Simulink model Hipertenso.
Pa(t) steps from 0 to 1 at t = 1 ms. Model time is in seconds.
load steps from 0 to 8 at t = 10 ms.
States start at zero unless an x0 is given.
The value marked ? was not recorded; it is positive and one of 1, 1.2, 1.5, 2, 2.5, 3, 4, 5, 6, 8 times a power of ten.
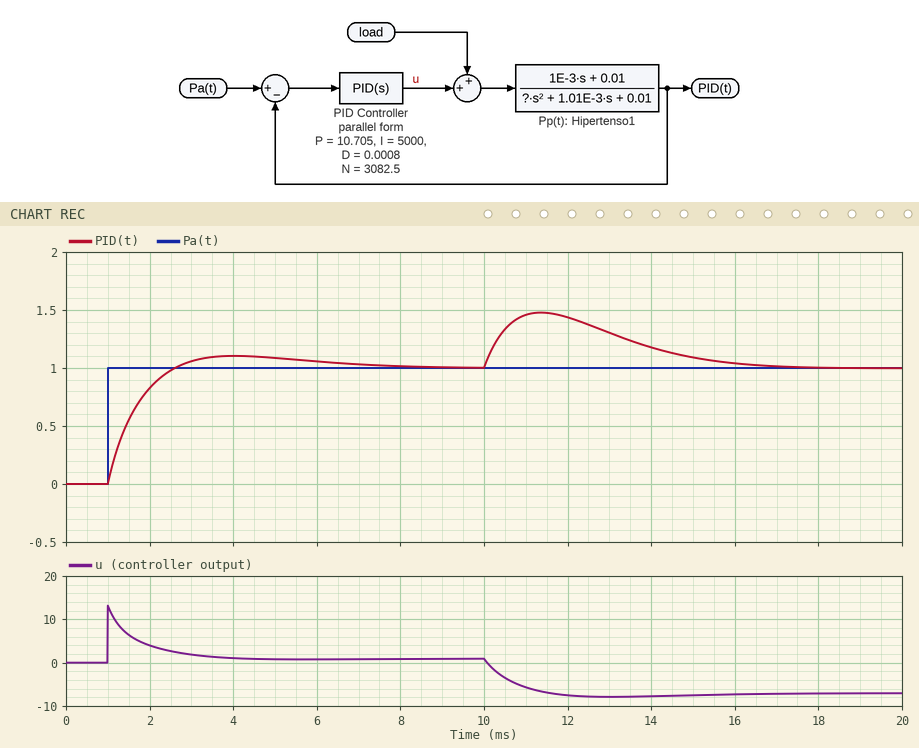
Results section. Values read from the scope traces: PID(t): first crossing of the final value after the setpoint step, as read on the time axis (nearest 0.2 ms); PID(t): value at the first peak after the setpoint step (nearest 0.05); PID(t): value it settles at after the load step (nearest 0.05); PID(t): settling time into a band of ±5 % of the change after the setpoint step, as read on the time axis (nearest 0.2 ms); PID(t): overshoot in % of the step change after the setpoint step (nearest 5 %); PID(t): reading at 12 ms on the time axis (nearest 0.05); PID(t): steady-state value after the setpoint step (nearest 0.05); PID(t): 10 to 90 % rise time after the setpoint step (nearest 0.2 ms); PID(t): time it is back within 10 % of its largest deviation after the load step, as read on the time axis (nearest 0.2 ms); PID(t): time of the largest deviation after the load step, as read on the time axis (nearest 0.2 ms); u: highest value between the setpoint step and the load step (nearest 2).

2.6 ms
1.10
1.00
6.2 ms
10 %
1.45
1.00
1.2 ms
15.8 ms
11.4 ms
14
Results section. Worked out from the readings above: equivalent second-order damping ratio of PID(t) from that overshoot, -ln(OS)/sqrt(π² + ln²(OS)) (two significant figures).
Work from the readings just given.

0.59
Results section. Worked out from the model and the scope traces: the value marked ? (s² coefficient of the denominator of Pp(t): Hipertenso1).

8e-06
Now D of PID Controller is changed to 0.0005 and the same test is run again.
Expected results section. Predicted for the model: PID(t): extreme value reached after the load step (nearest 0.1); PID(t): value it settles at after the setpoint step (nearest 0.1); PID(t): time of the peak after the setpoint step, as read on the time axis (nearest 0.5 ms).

1.5
1.0
4.0 ms
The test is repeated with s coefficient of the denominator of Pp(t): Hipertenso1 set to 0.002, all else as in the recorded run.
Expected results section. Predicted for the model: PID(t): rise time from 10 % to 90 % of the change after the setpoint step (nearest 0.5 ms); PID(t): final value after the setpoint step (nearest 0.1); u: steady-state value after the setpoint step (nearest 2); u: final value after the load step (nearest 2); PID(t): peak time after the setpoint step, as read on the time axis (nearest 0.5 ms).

1.5 ms
1.0
2
-6
4.5 ms
